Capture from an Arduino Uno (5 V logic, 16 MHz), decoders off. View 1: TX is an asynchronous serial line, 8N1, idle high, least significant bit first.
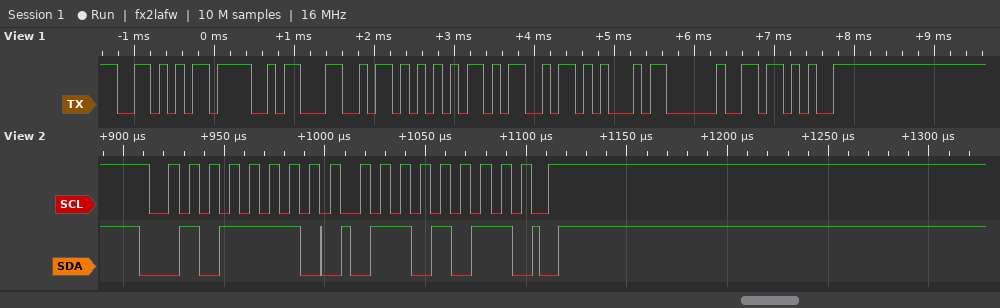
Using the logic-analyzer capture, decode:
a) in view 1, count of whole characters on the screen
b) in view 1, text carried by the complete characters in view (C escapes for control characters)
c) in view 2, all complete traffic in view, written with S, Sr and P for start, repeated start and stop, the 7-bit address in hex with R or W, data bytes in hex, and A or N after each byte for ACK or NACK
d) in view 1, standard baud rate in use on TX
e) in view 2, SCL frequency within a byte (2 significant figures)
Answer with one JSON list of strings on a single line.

["8", "\"VOLUME +\"", "S 2FW A 6B A P", "9600 baud", "100 kHz"]
